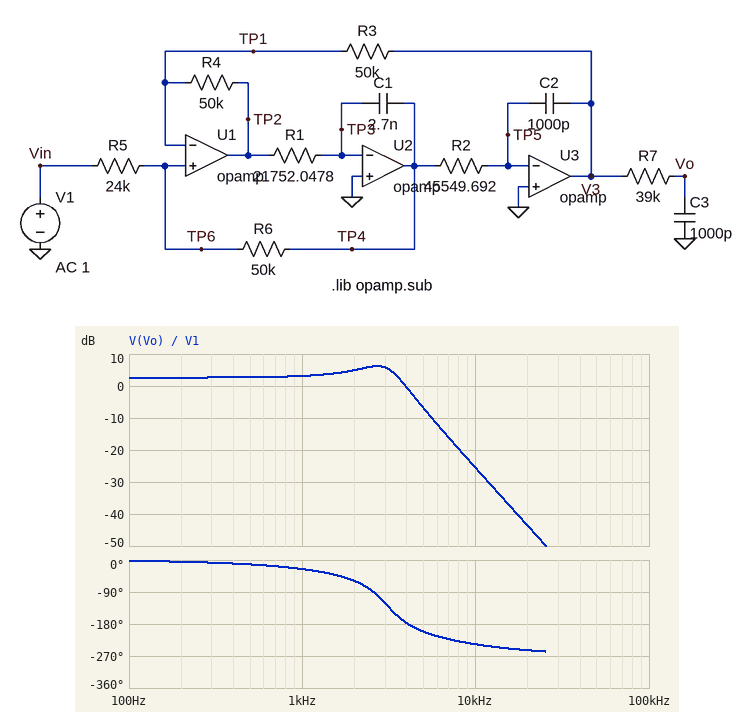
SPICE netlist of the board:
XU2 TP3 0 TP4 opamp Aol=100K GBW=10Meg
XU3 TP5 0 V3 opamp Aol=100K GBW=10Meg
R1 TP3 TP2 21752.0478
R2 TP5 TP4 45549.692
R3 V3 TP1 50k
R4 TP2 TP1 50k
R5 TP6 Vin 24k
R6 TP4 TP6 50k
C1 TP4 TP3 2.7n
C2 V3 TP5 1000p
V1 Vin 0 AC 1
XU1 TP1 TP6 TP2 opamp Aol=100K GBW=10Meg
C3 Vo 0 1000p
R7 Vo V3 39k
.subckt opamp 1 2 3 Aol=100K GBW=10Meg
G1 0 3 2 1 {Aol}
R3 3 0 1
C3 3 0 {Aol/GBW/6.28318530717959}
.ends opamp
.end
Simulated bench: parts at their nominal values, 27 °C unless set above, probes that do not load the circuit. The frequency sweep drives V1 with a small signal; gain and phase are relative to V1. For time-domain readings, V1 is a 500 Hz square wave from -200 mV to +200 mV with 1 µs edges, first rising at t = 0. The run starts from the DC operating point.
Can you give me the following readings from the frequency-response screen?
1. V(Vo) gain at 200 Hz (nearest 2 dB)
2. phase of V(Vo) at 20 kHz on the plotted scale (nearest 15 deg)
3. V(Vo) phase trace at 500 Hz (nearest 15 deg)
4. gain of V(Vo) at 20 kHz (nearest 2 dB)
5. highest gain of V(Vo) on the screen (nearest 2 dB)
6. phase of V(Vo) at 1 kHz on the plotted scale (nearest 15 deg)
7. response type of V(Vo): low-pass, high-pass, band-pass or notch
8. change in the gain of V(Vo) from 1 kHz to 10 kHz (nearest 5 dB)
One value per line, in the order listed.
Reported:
2 dB
-255 deg
-15 deg
-44 dB
6 dB
-30 deg
low-pass
-30 dB
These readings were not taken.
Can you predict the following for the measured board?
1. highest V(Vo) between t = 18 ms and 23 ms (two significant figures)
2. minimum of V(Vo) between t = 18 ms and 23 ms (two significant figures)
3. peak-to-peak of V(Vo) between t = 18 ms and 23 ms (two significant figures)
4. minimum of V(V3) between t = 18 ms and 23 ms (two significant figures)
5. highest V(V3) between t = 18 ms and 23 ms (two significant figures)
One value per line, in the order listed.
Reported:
430 mV
-430 mV
860 mV
-480 mV
480 mV
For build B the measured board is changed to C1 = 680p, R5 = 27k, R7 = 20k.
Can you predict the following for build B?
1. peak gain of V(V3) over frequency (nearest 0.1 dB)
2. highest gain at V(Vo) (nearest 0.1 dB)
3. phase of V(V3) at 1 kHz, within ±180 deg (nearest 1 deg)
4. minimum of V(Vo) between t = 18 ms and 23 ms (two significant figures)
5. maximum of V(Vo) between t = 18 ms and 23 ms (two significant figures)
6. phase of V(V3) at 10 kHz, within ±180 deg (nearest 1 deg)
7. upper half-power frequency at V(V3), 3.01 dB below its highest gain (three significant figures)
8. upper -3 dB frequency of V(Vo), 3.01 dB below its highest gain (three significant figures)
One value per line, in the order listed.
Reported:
2.5 dB
2.3 dB
-12 deg
-290 mV
290 mV
-130 deg
6.76 kHz
5.70 kHz
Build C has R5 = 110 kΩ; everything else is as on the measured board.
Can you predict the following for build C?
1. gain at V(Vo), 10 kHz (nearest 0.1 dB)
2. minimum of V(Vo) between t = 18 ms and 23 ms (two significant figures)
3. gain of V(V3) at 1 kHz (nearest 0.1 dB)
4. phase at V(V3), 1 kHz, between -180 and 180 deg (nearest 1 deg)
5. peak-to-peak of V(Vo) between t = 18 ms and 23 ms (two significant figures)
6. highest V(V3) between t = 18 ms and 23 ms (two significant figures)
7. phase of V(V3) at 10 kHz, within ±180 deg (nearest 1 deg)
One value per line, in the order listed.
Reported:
-32.8 dB
-140 mV
-3.9 dB
-24 deg
280 mV
150 mV
-158 deg
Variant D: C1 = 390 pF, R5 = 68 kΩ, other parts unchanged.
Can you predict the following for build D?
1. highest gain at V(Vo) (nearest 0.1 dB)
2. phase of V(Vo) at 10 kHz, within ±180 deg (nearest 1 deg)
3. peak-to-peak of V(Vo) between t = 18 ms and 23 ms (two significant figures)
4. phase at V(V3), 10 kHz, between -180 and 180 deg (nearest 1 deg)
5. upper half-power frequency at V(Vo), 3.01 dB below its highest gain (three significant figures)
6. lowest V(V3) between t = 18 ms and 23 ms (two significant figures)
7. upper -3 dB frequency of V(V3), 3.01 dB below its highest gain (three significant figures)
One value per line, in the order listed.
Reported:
-1.4 dB
-167 deg
340 mV
-99 deg
2.44 kHz
-170 mV
3.51 kHz
